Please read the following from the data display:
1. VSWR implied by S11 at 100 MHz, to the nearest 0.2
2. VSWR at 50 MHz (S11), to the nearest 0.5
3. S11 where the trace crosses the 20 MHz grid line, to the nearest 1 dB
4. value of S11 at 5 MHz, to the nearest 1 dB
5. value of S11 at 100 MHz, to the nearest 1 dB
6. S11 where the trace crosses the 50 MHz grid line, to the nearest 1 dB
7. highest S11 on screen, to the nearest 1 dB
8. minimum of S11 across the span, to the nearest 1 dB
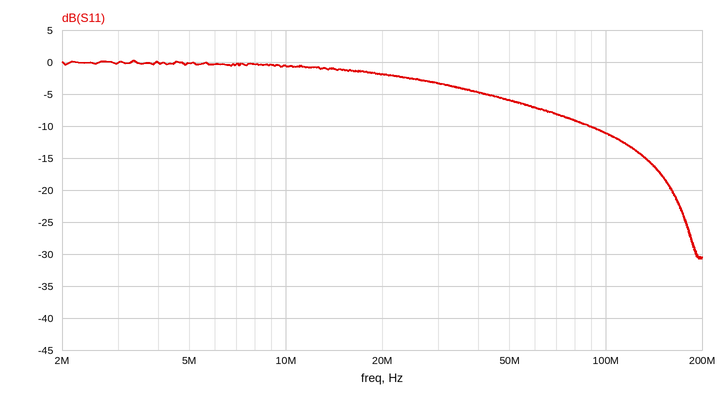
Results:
1.8
3.0
-2 dB
0 dB
-11 dB
-6 dB
0 dB
-31 dB
